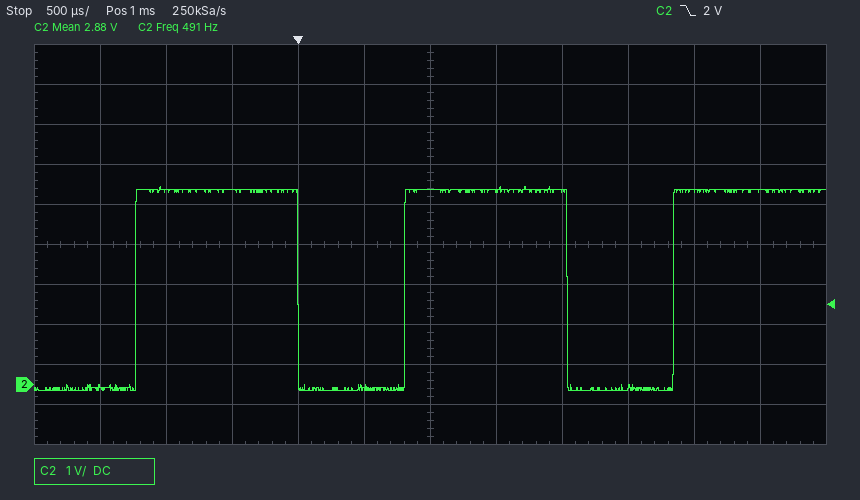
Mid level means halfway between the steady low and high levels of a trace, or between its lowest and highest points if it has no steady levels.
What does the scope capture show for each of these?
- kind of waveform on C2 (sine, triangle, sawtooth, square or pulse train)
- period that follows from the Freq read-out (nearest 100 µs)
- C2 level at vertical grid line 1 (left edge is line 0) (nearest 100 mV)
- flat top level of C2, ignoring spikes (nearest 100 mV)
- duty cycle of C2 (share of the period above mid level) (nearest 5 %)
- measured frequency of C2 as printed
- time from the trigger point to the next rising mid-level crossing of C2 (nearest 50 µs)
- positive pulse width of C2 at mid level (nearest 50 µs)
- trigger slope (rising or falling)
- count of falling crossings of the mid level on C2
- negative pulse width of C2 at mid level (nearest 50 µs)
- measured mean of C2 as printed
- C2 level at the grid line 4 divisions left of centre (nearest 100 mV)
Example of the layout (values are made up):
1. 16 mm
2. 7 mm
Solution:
1. pulse train
2. 2.0 ms
3. -100 mV
4. 4.9 V
5. 60 %
6. 491 Hz
7. 800 µs
8. 1.25 ms
9. falling
10. 2
11. 800 µs
12. 2.88 V
13. 4.8 V
